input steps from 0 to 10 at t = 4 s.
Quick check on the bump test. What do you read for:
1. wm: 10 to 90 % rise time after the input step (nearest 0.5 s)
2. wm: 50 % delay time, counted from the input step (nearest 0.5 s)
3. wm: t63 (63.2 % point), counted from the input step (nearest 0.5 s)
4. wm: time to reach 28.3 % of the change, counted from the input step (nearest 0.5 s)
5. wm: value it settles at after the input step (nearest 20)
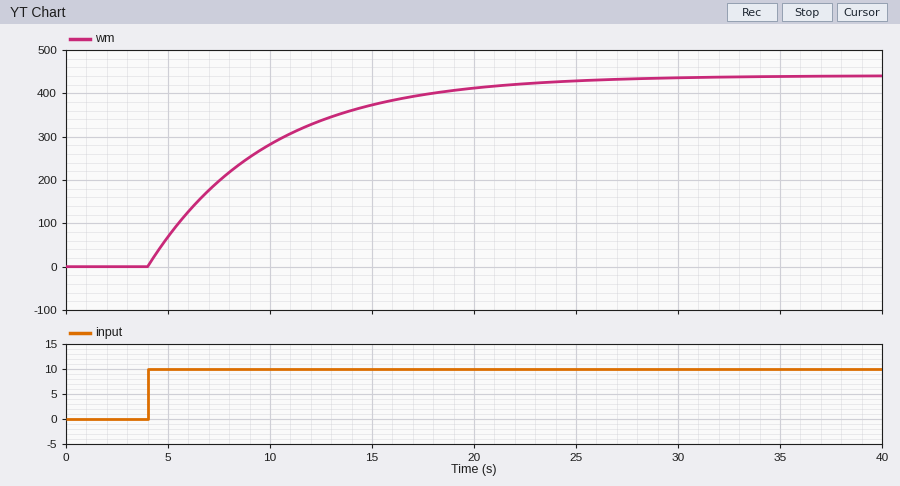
13.0 s
4.0 s
6.0 s
2.0 s
440
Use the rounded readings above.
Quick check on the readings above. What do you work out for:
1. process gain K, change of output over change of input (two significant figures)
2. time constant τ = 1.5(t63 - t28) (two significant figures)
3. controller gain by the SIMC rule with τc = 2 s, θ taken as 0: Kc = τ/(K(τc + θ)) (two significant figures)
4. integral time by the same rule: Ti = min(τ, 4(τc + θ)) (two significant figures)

44
6.0 s
0.068
6.0 s
